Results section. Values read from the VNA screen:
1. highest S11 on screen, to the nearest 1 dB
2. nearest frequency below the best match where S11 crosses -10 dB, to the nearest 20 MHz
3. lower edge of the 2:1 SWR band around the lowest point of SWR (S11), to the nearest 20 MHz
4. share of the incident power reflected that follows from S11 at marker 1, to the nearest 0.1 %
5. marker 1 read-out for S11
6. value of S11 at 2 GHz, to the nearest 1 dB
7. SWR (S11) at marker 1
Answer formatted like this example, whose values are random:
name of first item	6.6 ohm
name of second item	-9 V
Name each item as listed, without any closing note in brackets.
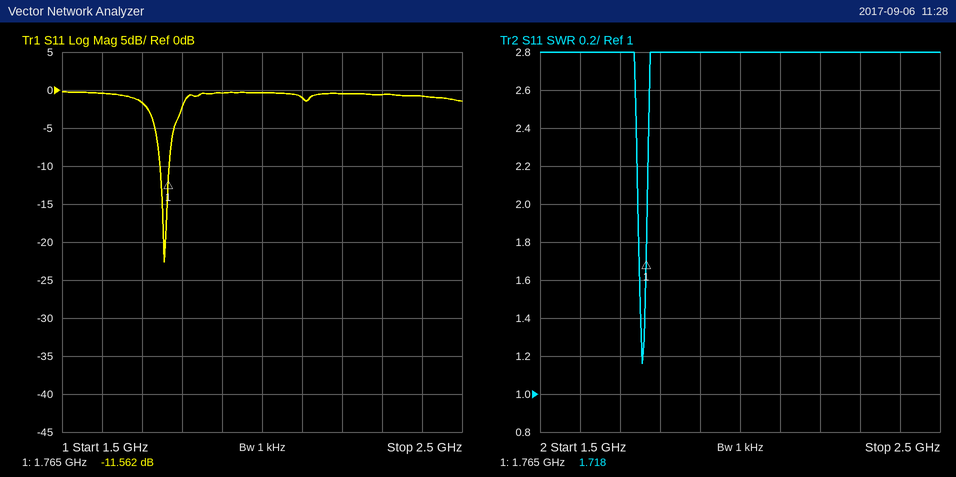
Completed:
highest S11 on screen, to the nearest 1 dB	0 dB
nearest frequency below the best match where S11 crosses -10 dB, to the nearest 20 MHz	1.74 GHz
lower edge of the 2:1 SWR band around the lowest point of SWR (S11), to the nearest 20 MHz	1.74 GHz
share of the incident power reflected that follows from S11 at marker 1, to the nearest 0.1 %	7.0 %
marker 1 read-out for S11	-11.562 dB
value of S11 at 2 GHz, to the nearest 1 dB	0 dB
SWR (S11) at marker 1	1.718
